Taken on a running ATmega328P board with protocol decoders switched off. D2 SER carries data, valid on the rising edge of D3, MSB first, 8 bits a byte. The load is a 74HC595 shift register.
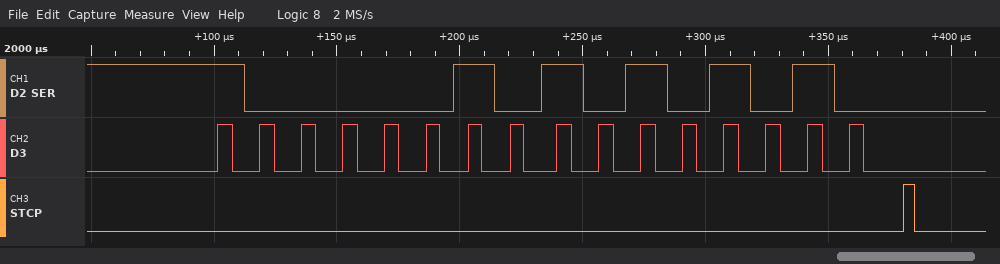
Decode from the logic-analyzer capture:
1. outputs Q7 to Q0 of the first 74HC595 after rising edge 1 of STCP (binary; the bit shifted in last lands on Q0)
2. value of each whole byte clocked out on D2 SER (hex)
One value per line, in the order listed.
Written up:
10101010
82 AA
